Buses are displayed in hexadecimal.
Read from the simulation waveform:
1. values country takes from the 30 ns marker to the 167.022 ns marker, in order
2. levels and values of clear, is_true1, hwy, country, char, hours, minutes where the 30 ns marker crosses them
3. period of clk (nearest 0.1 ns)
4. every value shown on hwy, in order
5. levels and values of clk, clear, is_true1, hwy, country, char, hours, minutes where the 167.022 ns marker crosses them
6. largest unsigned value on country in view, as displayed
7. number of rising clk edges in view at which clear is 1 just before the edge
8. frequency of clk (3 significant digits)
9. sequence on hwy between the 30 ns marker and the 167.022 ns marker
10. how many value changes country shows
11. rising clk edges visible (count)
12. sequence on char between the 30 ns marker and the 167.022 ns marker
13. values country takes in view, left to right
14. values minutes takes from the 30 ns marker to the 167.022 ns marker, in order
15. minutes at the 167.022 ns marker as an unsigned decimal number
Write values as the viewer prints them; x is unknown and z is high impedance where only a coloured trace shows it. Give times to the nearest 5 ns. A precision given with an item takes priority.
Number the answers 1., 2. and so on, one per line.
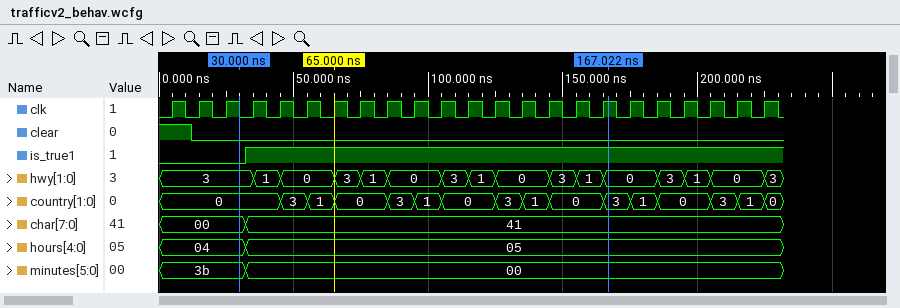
1. 0, 3, 1, 0, 3, 1, 0, 3, 1, 0, 3
2. clear=0, is_true1=0, hwy=3, country=0, char=00, hours=04, minutes=3b
3. 10 ns
4. 3, 1, 0, 3, 1, 0, 3, 1, 0, 3, 1, 0, 3, 1, 0, 3
5. clk=1, clear=0, is_true1=1, hwy=0, country=3, char=41, hours=05, minutes=00
6. 3
7. 1
8. 100 MHz
9. 3, 1, 0, 3, 1, 0, 3, 1, 0, 3, 1, 0
10. 15
11. 23
12. 00, 41
13. 0, 3, 1, 0, 3, 1, 0, 3, 1, 0, 3, 1, 0, 3, 1, 0
14. 3b, 00
15. 0
